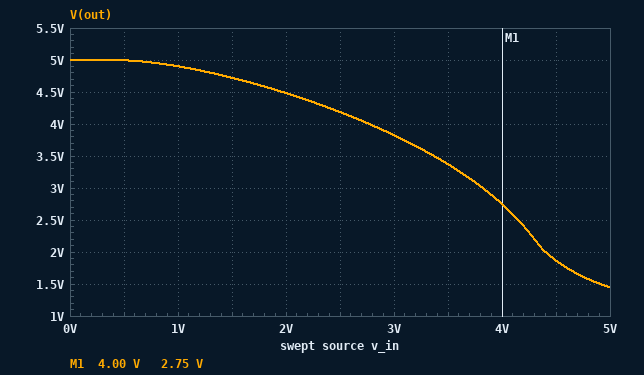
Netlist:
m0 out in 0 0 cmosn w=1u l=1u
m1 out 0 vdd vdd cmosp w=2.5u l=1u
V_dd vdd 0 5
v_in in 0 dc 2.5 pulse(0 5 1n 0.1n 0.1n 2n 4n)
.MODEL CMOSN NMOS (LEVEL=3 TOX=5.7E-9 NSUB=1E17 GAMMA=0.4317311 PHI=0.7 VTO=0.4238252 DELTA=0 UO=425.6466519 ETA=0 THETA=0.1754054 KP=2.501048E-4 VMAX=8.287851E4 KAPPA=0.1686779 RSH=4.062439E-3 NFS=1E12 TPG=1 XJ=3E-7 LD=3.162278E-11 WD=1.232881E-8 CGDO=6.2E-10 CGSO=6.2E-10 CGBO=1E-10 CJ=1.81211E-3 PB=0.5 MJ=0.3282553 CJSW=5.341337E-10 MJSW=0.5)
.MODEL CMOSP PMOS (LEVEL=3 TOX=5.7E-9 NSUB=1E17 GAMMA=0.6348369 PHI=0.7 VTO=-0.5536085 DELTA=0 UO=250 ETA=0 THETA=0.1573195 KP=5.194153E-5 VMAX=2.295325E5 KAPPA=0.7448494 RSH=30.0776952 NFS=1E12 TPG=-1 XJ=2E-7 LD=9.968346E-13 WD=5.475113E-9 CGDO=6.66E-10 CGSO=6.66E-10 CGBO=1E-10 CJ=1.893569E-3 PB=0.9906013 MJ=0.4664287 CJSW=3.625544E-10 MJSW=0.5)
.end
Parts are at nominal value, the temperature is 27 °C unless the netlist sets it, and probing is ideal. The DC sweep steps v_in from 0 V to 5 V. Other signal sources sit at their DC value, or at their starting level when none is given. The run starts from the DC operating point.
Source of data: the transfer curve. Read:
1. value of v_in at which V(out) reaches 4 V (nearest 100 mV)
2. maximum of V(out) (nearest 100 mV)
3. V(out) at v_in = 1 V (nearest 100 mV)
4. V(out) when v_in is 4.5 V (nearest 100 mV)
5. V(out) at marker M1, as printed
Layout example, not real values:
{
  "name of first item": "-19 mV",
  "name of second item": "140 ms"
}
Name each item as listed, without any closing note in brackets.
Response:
{
  "value of v_in at which V(out) reaches 4 V": "2.8 V",
  "maximum of V(out)": "5.0 V",
  "V(out) at v_in = 1 V": "4.9 V",
  "V(out) when v_in is 4.5 V": "1.9 V",
  "V(out) at marker M1, as printed": "2.75 V"
}
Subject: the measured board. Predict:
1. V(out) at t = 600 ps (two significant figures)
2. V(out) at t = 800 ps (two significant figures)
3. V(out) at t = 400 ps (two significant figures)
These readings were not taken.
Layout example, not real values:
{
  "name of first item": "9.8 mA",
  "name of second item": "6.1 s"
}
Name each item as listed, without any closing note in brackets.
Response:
{
  "V(out) at t = 600 ps": "5.0 V",
  "V(out) at t = 800 ps": "5.0 V",
  "V(out) at t = 400 ps": "5.0 V"
}
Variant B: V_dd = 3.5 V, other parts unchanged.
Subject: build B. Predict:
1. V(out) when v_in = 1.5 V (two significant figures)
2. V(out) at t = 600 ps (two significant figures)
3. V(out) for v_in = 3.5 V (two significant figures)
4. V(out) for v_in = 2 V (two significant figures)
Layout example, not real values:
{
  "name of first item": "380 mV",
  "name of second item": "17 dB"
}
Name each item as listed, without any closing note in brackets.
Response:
{
  "V(out) when v_in = 1.5 V": "3.1 V",
  "V(out) at t = 600 ps": "3.5 V",
  "V(out) for v_in = 3.5 V": "890 mV",
  "V(out) for v_in = 2 V": "2.8 V"
}
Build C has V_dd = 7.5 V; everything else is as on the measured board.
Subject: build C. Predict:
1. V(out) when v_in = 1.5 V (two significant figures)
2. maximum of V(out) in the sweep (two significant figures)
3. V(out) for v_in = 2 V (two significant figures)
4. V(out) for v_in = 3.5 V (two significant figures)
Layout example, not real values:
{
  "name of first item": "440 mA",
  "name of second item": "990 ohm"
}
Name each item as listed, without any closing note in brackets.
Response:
{
  "V(out) when v_in = 1.5 V": "7.3 V",
  "maximum of V(out) in the sweep": "7.5 V",
  "V(out) for v_in = 2 V": "7.1 V",
  "V(out) for v_in = 3.5 V": "6.4 V"
}
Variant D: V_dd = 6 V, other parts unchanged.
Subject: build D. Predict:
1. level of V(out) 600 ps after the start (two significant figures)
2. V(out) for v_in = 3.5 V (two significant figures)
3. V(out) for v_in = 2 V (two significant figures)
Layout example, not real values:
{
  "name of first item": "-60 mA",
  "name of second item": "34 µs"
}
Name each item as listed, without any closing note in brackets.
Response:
{
  "level of V(out) 600 ps after the start": "6.0 V",
  "V(out) for v_in = 3.5 V": "4.7 V",
  "V(out) for v_in = 2 V": "5.5 V"
}
